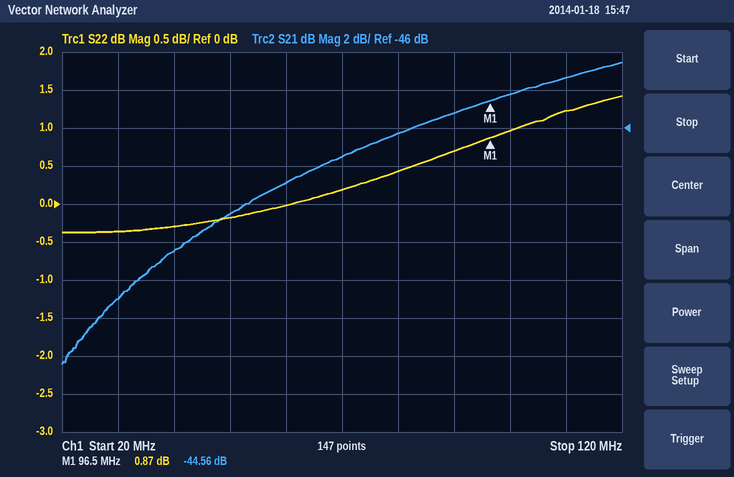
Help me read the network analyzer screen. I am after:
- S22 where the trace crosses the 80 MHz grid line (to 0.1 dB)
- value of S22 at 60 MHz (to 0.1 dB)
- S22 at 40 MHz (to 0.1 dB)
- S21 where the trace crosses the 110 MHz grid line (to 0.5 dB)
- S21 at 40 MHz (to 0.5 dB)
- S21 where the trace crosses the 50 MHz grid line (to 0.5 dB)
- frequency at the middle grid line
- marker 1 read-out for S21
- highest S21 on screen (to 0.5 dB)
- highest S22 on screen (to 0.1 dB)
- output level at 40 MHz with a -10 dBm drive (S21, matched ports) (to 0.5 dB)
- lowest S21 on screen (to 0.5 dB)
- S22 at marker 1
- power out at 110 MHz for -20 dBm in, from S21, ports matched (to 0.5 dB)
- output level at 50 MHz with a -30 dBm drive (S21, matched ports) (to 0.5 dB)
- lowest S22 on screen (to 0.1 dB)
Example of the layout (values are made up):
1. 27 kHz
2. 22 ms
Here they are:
1. 0.4 dB
2. 0.0 dB
3. -0.3 dB
4. -43.5 dB
5. -52.5 dB
6. -50.5 dB
7. 70 MHz
8. -44.56 dB
9. -42.5 dB
10. 1.4 dB
11. -62.5 dBm
12. -58.5 dB
13. 0.87 dB
14. -63.5 dBm
15. -80.5 dBm
16. -0.4 dB
